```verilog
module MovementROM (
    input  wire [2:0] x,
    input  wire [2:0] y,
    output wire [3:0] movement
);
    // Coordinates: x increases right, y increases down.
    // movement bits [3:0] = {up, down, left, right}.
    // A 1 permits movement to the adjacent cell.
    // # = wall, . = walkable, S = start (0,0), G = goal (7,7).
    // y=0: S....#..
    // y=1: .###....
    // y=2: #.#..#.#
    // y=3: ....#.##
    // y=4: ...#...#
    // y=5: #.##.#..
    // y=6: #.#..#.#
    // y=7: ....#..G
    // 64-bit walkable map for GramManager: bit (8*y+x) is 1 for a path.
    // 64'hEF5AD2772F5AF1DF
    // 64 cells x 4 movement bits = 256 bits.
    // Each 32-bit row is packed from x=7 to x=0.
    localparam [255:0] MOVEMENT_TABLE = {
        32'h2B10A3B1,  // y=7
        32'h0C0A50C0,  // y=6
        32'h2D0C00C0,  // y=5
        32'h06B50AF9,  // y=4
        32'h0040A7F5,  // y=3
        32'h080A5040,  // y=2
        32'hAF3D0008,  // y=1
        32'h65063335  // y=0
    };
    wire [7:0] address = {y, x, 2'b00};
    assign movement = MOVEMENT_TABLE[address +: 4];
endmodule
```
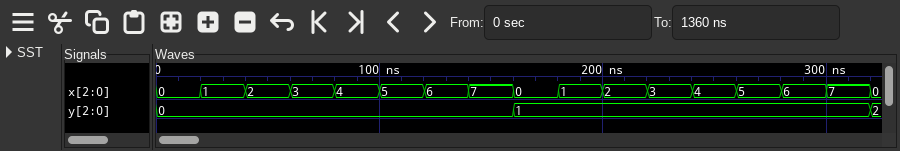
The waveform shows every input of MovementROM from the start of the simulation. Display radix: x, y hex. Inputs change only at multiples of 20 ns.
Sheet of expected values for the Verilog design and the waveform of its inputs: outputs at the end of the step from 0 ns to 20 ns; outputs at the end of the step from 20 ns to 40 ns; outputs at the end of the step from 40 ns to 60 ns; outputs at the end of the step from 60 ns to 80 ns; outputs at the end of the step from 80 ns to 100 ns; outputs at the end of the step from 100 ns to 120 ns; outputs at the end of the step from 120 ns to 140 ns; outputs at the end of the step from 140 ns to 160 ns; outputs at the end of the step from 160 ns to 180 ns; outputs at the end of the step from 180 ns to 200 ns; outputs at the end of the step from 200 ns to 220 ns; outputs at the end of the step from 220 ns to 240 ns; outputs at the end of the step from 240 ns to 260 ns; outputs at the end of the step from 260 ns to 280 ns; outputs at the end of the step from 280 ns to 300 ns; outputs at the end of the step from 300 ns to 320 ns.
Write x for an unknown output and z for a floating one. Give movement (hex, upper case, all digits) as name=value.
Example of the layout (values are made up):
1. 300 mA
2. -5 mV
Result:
1. movement=5
2. movement=3
3. movement=3
4. movement=3
5. movement=6
6. movement=0
7. movement=5
8. movement=6
9. movement=8
10. movement=0
11. movement=0
12. movement=0
13. movement=D
14. movement=3
15. movement=F
16. movement=A
